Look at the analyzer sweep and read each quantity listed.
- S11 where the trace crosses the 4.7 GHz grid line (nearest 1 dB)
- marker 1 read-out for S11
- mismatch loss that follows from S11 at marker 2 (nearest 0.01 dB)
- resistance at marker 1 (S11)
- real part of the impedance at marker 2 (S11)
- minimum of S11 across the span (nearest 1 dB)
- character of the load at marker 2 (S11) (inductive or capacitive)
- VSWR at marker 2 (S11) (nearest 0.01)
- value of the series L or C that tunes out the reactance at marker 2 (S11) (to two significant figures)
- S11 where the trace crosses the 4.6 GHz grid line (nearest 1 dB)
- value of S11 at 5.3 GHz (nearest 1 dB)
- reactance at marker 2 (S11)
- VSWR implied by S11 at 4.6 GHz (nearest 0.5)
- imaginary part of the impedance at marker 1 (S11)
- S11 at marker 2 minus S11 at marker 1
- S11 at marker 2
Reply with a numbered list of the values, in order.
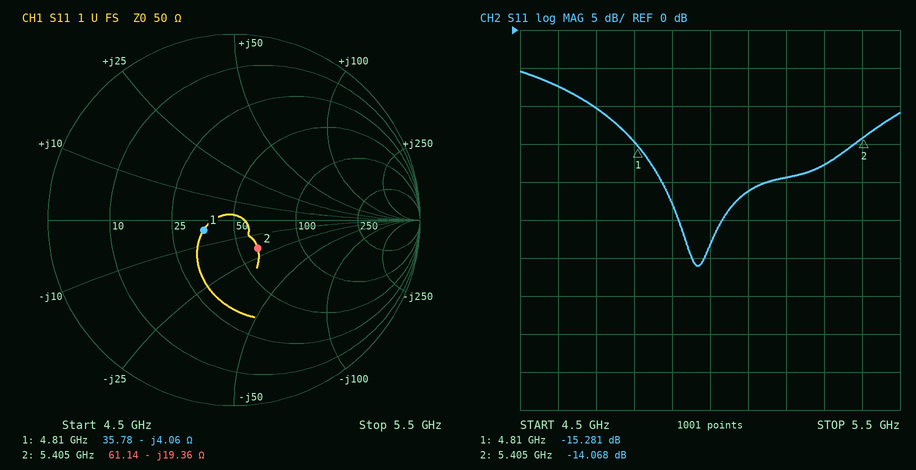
1. -10 dB
2. -15.281 dB
3. 0.17 dB
4. 35.78 Ω
5. 61.14 Ω
6. -31 dB
7. capacitive
8. 1.49
9. 570 pH
10. -7 dB
11. -18 dB
12. -19.36 Ω
13. 2.5
14. -4.06 Ω
15. 1.213 dB
16. -14.068 dB
